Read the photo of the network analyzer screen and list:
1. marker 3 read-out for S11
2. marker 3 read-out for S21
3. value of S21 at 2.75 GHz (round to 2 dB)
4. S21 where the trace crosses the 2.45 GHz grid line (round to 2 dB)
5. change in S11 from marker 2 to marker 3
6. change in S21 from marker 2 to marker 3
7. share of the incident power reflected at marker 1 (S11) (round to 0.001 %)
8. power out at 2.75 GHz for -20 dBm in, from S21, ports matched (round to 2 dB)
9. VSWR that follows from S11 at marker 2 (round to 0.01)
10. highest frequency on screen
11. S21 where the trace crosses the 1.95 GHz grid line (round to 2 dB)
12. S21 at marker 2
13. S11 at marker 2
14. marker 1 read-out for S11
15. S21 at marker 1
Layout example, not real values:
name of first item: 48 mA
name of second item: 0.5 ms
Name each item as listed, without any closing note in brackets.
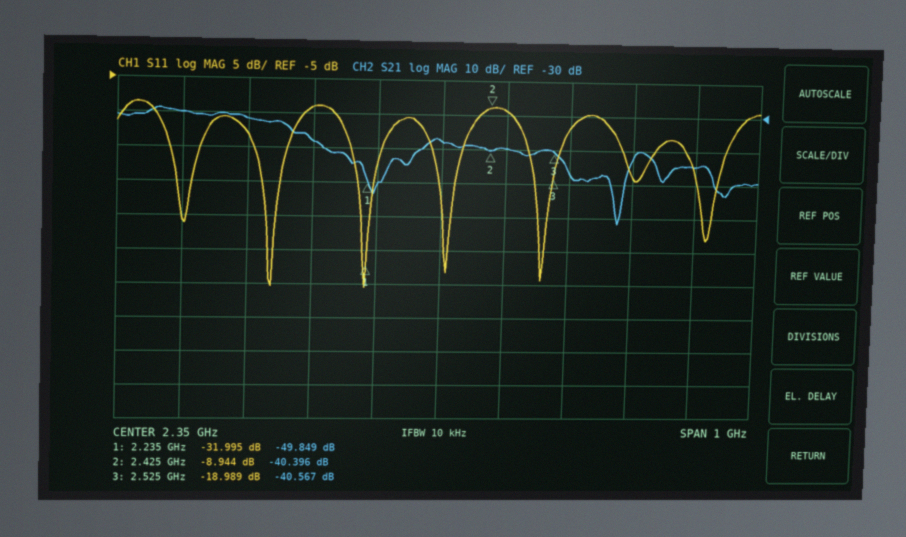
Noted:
marker 3 read-out for S11: -18.989 dB
marker 3 read-out for S21: -40.567 dB
value of S21 at 2.75 GHz: -44 dB
S21 where the trace crosses the 2.45 GHz grid line: -40 dB
change in S11 from marker 2 to marker 3: -10.045 dB
change in S21 from marker 2 to marker 3: -0.171 dB
share of the incident power reflected at marker 1 (S11): 0.063 %
power out at 2.75 GHz for -20 dBm in, from S21, ports matched: -64 dBm
VSWR that follows from S11 at marker 2: 2.11
highest frequency on screen: 2.85 GHz
S21 where the trace crosses the 1.95 GHz grid line: -30 dB
S21 at marker 2: -40.396 dB
S11 at marker 2: -8.944 dB
marker 1 read-out for S11: -31.995 dB
S21 at marker 1: -49.849 dB
